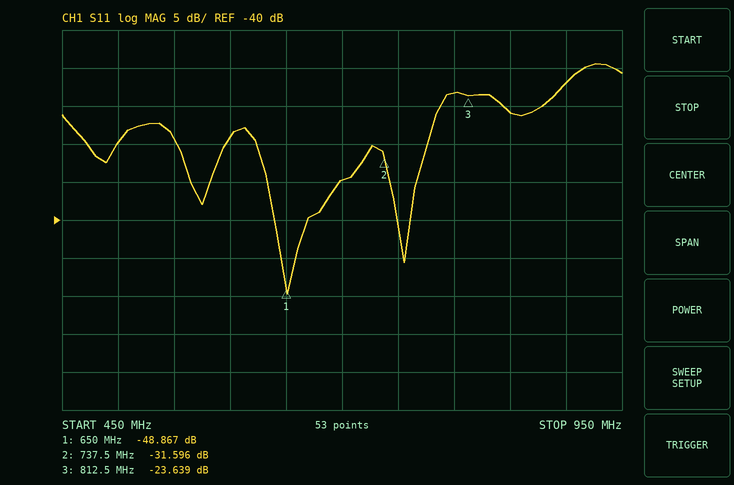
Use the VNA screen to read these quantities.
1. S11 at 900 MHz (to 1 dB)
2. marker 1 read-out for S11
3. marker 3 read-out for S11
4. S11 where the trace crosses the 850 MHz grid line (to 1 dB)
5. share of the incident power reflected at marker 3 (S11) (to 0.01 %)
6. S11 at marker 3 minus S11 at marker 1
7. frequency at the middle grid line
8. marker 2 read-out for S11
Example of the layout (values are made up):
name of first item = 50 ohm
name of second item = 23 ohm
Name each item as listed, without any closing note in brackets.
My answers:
S11 at 900 MHz = -22 dB
marker 1 read-out for S11 = -48.867 dB
marker 3 read-out for S11 = -23.639 dB
S11 where the trace crosses the 850 MHz grid line = -26 dB
share of the incident power reflected at marker 3 (S11) = 0.43 %
S11 at marker 3 minus S11 at marker 1 = 25.228 dB
frequency at the middle grid line = 700 MHz
marker 2 read-out for S11 = -31.596 dB
